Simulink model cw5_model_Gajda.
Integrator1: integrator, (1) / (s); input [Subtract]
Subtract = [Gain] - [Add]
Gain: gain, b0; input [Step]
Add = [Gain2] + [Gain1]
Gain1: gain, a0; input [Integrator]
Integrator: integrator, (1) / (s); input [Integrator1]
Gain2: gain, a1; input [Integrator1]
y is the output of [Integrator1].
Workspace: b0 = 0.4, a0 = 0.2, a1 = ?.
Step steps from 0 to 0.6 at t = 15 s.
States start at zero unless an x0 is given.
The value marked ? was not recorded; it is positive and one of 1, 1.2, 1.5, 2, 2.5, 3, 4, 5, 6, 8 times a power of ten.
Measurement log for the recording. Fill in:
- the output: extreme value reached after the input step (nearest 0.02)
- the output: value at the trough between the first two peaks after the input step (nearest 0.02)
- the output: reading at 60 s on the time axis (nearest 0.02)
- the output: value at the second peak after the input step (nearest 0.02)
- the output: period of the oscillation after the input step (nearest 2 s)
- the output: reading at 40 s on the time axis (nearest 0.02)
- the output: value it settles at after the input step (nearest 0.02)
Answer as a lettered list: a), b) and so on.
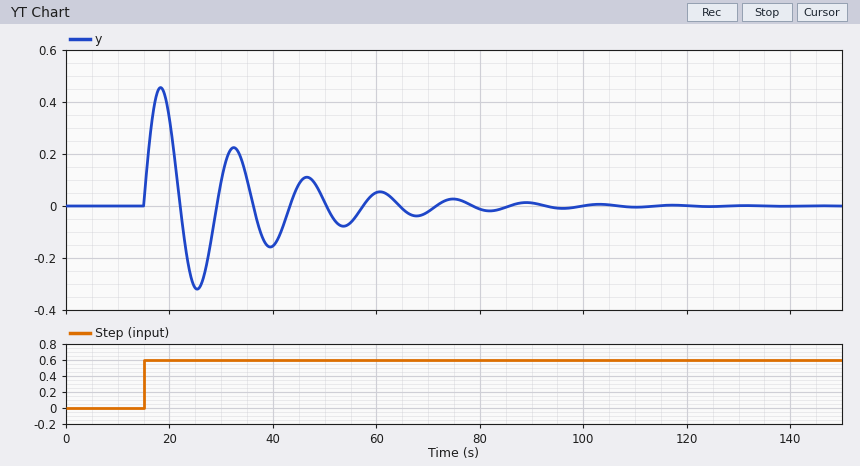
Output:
a) 0.46
b) -0.32
c) 0.06
d) 0.22
e) 14 s
f) -0.16
g) 0.00
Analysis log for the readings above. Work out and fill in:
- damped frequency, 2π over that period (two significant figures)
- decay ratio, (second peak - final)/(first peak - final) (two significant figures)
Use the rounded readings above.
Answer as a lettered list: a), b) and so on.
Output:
a) 0.45 rad/s
b) 0.48
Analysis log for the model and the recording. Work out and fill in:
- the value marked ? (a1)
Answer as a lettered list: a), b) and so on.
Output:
a) 0.1
